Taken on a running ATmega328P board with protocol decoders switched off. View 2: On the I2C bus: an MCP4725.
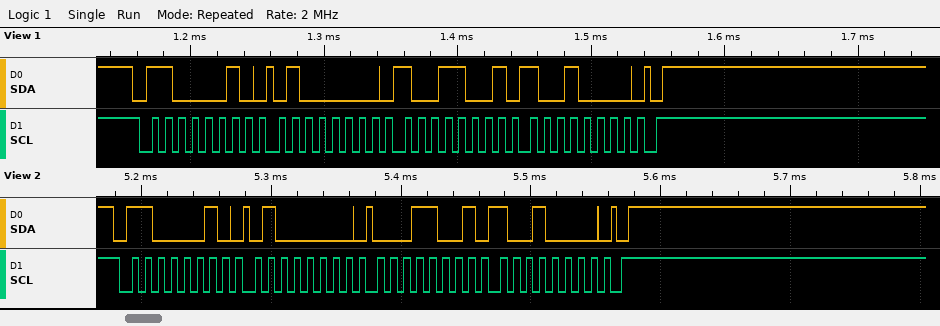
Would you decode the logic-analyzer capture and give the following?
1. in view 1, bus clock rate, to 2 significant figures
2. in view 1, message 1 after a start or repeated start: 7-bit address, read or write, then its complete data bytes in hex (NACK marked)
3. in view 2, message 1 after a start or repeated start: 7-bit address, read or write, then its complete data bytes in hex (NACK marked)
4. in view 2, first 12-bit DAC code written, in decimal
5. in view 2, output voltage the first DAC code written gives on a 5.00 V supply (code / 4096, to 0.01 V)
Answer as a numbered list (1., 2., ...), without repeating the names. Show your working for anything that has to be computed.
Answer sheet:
1. 100 kHz
2. 0x61 write: 40 99 90
3. 0x61 write: 40 19 90
4. 409
5. 409 / 4096 x 5.00 V = 0.50 V
